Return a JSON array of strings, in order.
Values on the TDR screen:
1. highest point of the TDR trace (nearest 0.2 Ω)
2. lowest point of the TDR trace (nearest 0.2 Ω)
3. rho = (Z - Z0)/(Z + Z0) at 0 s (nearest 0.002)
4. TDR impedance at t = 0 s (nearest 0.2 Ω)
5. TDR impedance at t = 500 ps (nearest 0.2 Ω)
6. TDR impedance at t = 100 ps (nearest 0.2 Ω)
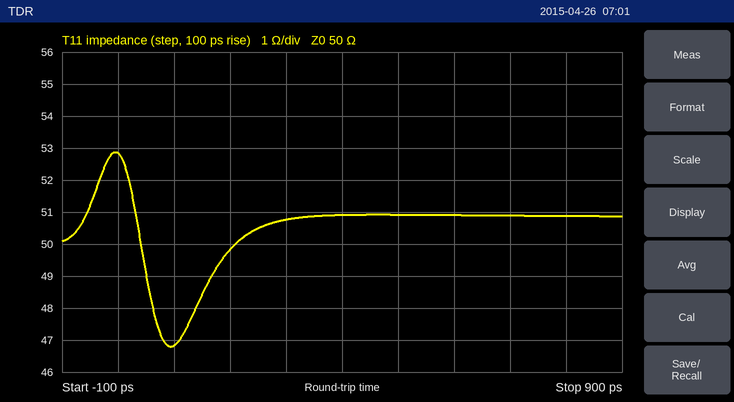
["52.8 Ω", "46.8 Ω", "+0.028", "52.8 Ω", "51.0 Ω", "46.8 Ω"]
